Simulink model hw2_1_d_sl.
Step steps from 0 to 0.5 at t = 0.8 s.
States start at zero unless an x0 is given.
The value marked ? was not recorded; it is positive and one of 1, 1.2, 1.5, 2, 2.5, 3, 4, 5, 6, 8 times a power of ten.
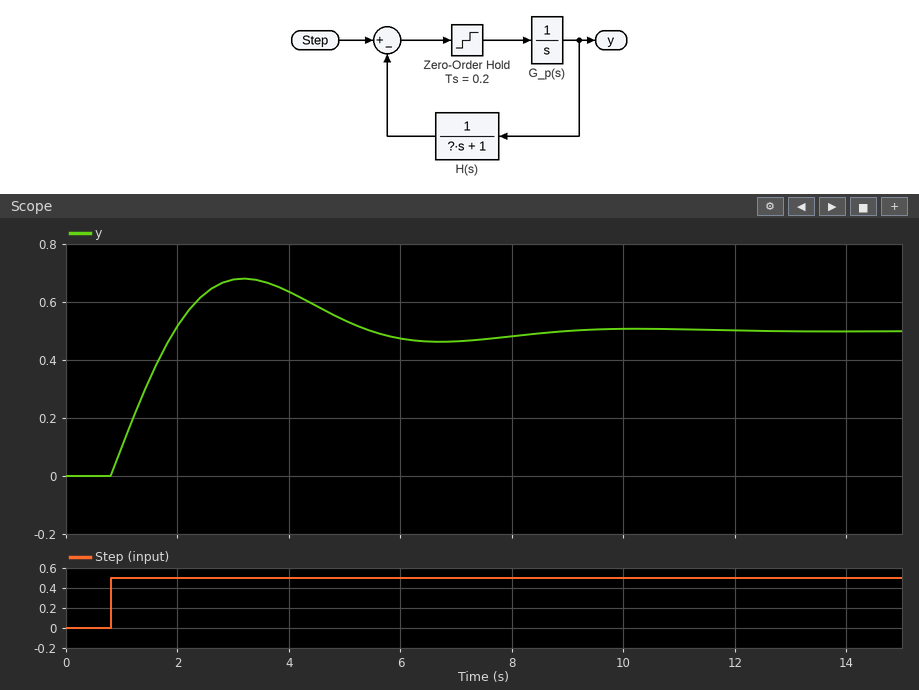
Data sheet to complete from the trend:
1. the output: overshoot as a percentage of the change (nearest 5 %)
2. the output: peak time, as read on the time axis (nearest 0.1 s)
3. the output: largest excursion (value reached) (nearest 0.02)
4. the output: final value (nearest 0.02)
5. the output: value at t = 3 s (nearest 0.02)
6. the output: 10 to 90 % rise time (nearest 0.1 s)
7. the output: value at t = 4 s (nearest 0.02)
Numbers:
35 %
3.2 s
0.68
0.50
0.68
0.9 s
0.64
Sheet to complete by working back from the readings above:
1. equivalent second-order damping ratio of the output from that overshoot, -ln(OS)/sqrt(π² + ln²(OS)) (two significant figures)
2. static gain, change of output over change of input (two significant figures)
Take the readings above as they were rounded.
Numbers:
0.32
1.0
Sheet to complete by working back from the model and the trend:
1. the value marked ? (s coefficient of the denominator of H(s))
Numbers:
1
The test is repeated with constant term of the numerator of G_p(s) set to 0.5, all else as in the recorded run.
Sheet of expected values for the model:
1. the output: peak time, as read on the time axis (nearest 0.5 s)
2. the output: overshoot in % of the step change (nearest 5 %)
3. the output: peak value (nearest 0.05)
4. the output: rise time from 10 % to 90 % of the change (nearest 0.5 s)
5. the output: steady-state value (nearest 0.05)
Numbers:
5.5 s
10 %
0.55
2.0 s
0.50
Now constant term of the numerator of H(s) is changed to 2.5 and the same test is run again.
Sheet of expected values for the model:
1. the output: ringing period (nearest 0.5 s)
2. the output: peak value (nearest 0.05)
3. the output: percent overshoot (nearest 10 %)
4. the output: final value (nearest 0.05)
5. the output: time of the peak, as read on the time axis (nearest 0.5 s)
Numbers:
4.0 s
0.40
100 %
0.20
2.0 s
